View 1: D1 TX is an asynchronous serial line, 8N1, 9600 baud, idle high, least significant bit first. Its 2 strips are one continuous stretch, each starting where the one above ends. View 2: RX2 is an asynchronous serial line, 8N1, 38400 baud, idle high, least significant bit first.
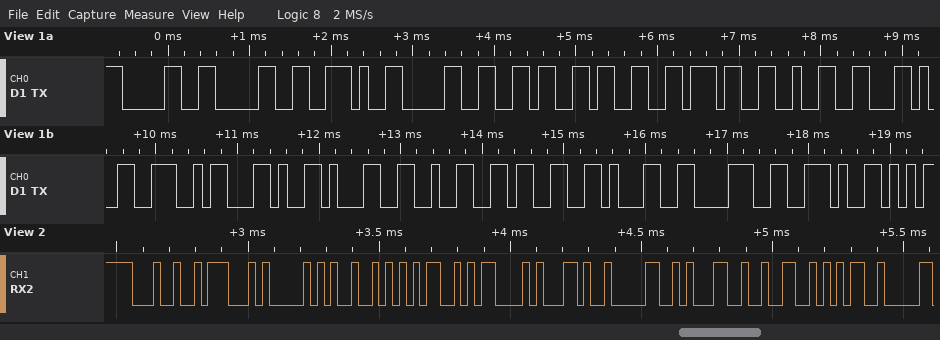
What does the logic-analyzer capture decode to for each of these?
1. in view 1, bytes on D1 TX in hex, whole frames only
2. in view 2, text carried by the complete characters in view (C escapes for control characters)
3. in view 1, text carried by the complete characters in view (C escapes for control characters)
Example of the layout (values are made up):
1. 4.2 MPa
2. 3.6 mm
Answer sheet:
1. 30 30 2E 30 36 33 37 32 2C 4E 2C 31 32 33 31 38 2E
2. "$GPRMC,0125"
3. "00.06372,N,12318."
